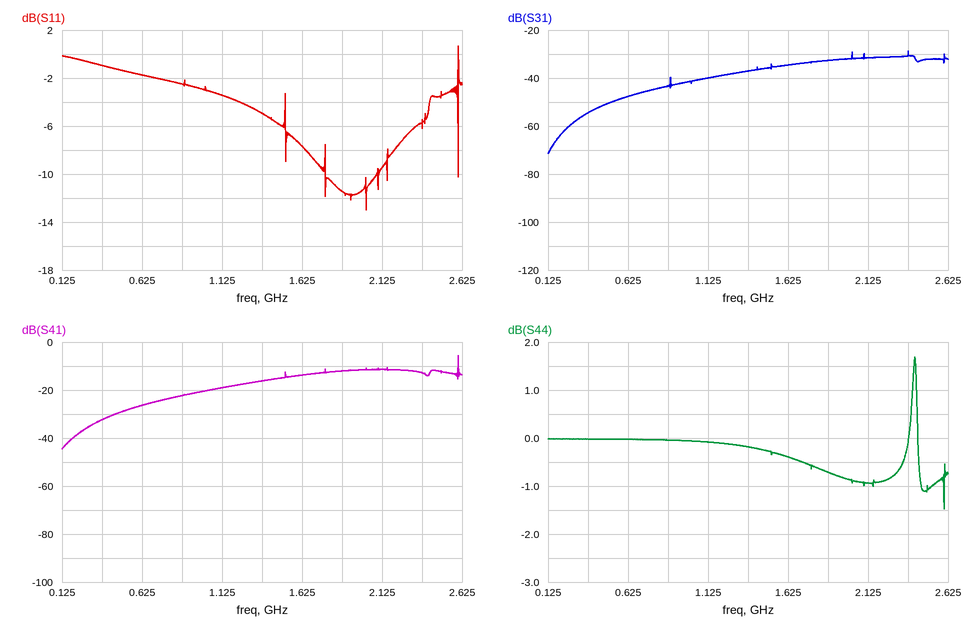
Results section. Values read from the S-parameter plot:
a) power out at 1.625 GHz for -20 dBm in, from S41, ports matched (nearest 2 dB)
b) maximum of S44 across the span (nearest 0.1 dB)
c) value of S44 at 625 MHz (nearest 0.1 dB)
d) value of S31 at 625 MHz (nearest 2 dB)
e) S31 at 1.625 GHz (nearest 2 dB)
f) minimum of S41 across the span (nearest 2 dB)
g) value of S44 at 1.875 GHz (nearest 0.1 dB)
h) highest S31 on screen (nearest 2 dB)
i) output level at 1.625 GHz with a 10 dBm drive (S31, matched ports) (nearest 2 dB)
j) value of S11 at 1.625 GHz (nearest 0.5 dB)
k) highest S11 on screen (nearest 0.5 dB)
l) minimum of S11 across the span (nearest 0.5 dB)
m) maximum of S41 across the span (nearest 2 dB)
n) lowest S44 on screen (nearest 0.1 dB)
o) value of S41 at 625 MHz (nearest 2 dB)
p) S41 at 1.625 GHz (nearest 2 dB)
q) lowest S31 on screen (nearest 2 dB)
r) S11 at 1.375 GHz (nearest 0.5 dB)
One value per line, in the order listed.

-34 dBm
1.7 dB
0.0 dB
-48 dB
-34 dB
-44 dB
-0.7 dB
-28 dB
-24 dBm
-7.5 dB
0.5 dB
-13.0 dB
-6 dB
-1.5 dB
-26 dB
-14 dB
-72 dB
-5.0 dB
